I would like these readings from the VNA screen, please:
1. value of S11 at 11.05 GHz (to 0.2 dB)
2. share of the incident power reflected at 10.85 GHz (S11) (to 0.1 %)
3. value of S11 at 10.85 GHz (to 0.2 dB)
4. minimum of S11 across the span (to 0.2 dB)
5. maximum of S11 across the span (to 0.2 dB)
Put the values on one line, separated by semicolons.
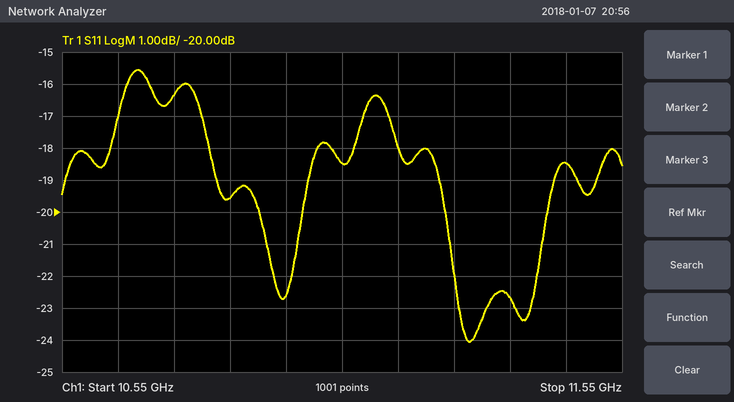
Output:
-18.4 dB; 1.1 %; -19.6 dB; -24.0 dB; -15.6 dB
